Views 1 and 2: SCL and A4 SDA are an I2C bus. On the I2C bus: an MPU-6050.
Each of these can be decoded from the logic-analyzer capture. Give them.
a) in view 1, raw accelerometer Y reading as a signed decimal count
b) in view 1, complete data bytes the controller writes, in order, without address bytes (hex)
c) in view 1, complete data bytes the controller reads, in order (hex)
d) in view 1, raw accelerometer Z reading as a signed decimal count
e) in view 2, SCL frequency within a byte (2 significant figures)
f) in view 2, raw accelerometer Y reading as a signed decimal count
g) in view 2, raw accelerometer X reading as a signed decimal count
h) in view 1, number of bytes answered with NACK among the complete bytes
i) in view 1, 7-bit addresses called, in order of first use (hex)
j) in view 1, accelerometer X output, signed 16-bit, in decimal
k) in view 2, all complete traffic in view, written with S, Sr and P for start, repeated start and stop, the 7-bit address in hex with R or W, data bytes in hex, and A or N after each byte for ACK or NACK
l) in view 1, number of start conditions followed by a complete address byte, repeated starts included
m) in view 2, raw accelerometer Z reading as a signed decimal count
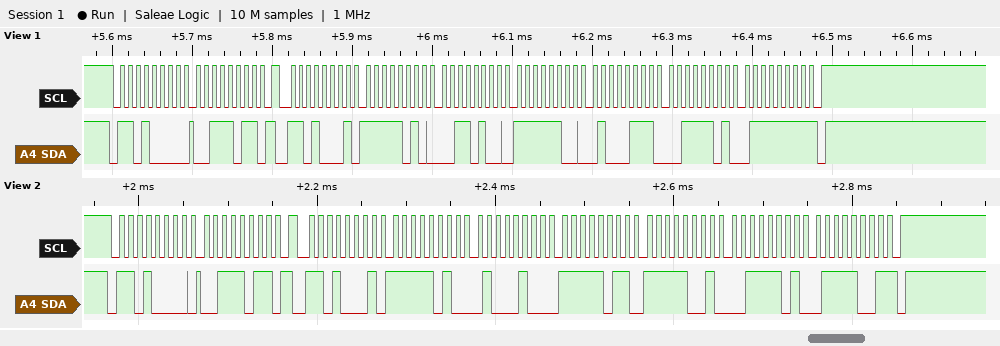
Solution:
-953
3B
FA 34 FC 47 3D 7F
15743
100 kHz
-1031
-1468
1
0x68
-1484
S 68W A 3B A Sr 68R A FA A 44 A FB A F9 A 3D A 79 N P
2
15737
